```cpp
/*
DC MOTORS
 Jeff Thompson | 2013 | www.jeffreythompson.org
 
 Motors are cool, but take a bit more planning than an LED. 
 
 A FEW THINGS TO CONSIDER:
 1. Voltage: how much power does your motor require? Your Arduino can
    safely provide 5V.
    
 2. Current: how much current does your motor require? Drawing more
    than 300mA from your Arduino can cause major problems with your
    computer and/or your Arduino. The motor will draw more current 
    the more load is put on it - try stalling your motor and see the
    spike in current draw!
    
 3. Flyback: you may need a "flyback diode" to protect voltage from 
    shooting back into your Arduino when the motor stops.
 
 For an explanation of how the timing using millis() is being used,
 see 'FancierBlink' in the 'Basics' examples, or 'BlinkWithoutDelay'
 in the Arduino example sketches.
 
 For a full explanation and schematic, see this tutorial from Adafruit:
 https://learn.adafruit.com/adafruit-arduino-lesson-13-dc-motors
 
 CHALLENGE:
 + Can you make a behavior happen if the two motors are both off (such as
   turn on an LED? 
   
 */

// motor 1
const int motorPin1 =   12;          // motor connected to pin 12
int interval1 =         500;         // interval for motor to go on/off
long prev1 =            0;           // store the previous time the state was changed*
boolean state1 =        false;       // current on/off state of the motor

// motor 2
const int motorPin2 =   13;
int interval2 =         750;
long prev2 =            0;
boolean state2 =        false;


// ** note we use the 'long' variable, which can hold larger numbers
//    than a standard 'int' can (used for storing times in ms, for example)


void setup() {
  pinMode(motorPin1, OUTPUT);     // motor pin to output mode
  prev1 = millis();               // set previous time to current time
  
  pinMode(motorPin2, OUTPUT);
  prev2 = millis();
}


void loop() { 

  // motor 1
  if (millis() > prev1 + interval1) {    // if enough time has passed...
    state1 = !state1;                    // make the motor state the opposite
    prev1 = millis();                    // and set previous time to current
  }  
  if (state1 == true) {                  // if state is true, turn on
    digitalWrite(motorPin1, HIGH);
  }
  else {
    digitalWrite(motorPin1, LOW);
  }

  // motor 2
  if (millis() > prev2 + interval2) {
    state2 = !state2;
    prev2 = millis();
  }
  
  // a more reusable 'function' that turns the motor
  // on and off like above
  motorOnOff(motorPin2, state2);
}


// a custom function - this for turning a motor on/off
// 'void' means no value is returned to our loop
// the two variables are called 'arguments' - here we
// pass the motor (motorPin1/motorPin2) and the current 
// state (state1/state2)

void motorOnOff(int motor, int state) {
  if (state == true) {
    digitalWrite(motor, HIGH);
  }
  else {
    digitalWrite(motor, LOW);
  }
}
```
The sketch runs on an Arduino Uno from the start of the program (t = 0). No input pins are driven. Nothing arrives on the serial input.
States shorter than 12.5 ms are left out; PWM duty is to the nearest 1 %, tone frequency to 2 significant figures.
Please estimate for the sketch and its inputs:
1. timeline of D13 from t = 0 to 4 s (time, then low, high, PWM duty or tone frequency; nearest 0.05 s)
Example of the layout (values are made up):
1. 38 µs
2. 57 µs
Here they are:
1. 0 s low; 0.75 s high; 1.5 s low; 2.25 s high; 3 s low; 3.75 s high
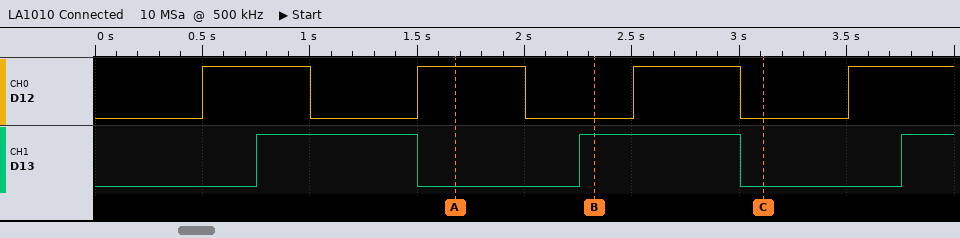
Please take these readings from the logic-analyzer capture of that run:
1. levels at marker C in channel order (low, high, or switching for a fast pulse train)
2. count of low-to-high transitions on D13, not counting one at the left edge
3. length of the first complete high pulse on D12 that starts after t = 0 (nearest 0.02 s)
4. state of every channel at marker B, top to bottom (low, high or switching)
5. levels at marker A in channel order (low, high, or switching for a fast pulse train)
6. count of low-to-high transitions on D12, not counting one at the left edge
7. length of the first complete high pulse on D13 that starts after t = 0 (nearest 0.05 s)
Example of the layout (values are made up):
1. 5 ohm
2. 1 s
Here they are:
1. D12 low, D13 low
2. 3
3. 0.50 s
4. D12 low, D13 high
5. D12 high, D13 low
6. 4
7. 0.75 s
